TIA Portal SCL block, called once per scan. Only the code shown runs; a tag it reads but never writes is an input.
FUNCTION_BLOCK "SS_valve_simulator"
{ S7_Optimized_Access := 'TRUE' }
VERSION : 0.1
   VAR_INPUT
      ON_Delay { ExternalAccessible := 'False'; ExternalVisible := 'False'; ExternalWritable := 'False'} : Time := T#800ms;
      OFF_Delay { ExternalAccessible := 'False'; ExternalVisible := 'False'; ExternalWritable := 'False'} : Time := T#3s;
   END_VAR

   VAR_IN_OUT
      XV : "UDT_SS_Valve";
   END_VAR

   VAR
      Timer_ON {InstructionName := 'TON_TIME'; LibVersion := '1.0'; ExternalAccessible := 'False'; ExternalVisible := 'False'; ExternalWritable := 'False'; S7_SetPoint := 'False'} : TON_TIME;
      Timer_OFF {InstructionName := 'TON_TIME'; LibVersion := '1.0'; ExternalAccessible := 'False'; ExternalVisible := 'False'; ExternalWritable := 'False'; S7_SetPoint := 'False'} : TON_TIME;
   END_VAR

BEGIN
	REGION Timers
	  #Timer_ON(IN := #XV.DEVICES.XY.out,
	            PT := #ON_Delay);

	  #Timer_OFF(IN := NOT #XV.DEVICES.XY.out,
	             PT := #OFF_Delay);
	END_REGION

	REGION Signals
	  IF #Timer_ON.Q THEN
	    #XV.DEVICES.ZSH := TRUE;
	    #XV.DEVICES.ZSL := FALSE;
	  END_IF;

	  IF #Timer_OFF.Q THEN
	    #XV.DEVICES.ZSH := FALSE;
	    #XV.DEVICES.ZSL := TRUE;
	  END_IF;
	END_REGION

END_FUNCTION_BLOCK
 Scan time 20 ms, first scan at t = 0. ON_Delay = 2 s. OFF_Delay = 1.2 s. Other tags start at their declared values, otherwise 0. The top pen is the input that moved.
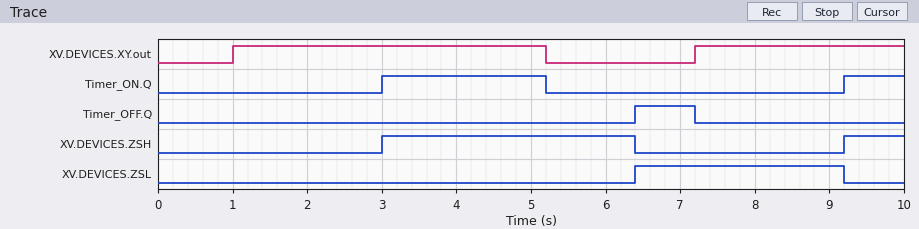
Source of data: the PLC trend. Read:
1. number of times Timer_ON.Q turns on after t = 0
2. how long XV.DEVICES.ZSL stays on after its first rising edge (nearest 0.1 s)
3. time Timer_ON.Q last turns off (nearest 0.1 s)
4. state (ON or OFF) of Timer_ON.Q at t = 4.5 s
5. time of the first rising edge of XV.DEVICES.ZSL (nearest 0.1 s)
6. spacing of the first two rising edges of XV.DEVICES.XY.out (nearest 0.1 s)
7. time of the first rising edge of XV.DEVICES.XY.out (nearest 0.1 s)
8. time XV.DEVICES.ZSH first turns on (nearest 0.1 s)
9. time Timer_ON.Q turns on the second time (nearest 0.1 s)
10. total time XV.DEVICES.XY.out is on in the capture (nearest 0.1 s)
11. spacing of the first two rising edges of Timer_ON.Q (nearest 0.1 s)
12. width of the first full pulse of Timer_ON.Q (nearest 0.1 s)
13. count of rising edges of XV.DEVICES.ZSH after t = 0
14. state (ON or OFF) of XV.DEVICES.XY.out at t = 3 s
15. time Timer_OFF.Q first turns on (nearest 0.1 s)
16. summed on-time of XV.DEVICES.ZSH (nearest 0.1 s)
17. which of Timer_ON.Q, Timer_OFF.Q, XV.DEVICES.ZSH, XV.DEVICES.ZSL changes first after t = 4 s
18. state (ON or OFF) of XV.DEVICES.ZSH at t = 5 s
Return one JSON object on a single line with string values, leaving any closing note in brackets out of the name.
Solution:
{"number of times Timer_ON.Q turns on after t = 0": "2", "how long XV.DEVICES.ZSL stays on after its first rising edge": "2.8 s", "time Timer_ON.Q last turns off": "5.2 s", "state (ON or OFF) of Timer_ON.Q at t = 4.5 s": "ON", "time of the first rising edge of XV.DEVICES.ZSL": "6.4 s", "spacing of the first two rising edges of XV.DEVICES.XY.out": "6.2 s", "time of the first rising edge of XV.DEVICES.XY.out": "1.0 s", "time XV.DEVICES.ZSH first turns on": "3.0 s", "time Timer_ON.Q turns on the second time": "9.2 s", "total time XV.DEVICES.XY.out is on in the capture": "7.0 s", "spacing of the first two rising edges of Timer_ON.Q": "6.2 s", "width of the first full pulse of Timer_ON.Q": "2.2 s", "count of rising edges of XV.DEVICES.ZSH after t = 0": "2", "state (ON or OFF) of XV.DEVICES.XY.out at t = 3 s": "ON", "time Timer_OFF.Q first turns on": "6.4 s", "summed on-time of XV.DEVICES.ZSH": "4.2 s", "which of Timer_ON.Q, Timer_OFF.Q, XV.DEVICES.ZSH, XV.DEVICES.ZSL changes first after t = 4 s": "Timer_ON.Q", "state (ON or OFF) of XV.DEVICES.ZSH at t = 5 s": "ON"}
